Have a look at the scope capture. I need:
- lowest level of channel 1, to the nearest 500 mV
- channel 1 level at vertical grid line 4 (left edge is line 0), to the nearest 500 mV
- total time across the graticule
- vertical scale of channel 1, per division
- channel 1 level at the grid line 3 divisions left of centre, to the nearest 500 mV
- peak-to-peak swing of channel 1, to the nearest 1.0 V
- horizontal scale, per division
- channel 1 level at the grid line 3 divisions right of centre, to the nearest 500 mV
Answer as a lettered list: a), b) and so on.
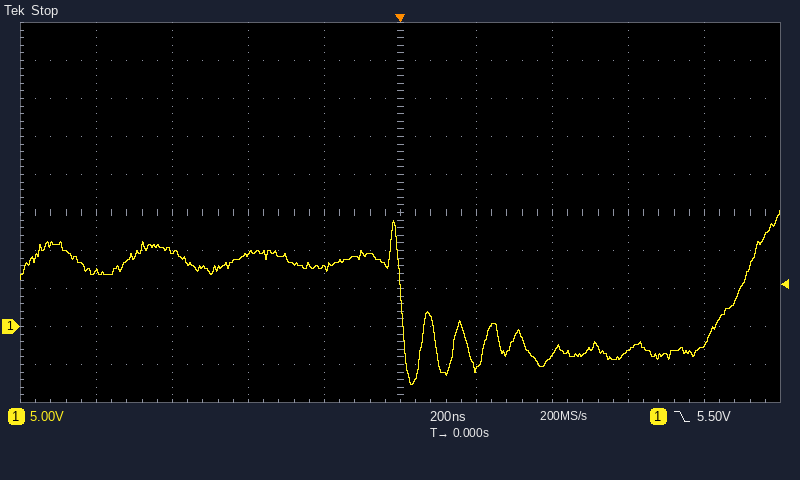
a) -7.5 V
b) 7.5 V
c) 2 µs
d) 5 V
e) 10.0 V
f) 23.0 V
g) 200 ns
h) -3.0 V
